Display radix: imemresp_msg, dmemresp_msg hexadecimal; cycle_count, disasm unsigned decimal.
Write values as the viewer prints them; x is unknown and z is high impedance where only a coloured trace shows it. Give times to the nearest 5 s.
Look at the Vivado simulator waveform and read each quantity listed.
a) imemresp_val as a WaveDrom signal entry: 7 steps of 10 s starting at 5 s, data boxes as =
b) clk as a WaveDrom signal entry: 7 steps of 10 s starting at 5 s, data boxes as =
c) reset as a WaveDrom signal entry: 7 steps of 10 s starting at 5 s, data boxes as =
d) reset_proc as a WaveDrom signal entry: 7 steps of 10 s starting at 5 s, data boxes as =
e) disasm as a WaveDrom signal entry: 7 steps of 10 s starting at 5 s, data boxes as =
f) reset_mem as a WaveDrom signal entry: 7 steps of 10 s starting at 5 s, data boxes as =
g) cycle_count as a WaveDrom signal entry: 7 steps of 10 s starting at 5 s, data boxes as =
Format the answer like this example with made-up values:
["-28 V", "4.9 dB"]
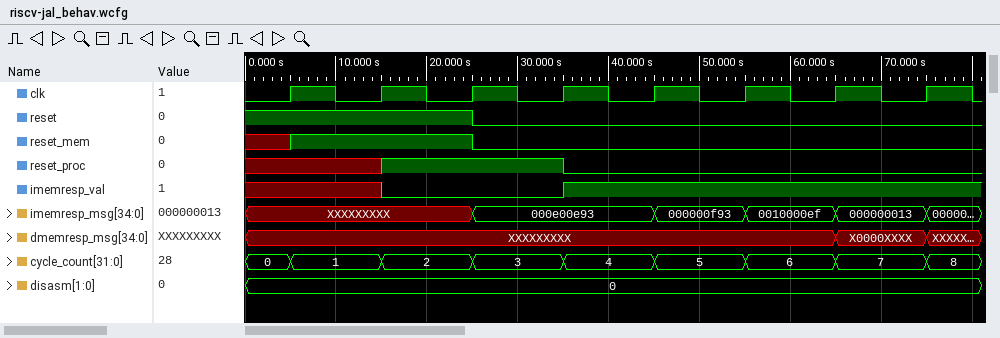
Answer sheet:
["{name: 'imemresp_val', wave: 'x0.1...'}", "{name: 'clk', wave: 'p......'}", "{name: 'reset', wave: '1.0....'}", "{name: 'reset_proc', wave: 'x1.0...'}", "{name: 'disasm', wave: '=......', data: '0'}", "{name: 'reset_mem', wave: '1.0....'}", "{name: 'cycle_count', wave: '=======', data: '1 2 3 4 5 6 7'}"]
